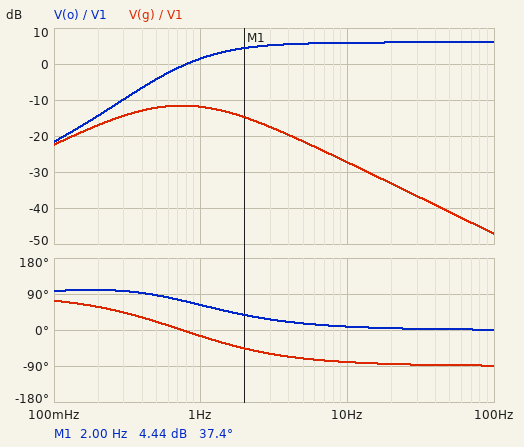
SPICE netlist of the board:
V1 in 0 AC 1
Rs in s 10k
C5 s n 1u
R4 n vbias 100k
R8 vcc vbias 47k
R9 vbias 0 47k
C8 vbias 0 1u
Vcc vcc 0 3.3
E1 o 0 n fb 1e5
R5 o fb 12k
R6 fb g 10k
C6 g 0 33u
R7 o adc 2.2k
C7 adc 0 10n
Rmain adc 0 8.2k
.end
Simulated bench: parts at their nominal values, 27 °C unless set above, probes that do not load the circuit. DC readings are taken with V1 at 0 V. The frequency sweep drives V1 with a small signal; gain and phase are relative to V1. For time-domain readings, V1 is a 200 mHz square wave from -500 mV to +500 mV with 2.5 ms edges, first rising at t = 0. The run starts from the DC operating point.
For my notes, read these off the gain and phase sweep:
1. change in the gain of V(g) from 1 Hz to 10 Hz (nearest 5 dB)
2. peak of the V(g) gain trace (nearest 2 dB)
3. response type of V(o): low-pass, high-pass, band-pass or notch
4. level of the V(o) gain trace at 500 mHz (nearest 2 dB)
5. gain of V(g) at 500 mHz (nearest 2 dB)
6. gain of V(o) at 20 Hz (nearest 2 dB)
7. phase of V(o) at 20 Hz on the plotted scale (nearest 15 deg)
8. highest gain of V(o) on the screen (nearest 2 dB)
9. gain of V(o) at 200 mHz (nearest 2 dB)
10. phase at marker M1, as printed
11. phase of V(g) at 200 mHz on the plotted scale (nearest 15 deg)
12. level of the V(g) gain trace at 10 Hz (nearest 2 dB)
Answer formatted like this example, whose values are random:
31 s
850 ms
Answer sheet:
-15 dB
-12 dB
high-pass
-4 dB
-12 dB
6 dB
0 deg
6 dB
-14 dB
37.4 deg
60 deg
-28 dB
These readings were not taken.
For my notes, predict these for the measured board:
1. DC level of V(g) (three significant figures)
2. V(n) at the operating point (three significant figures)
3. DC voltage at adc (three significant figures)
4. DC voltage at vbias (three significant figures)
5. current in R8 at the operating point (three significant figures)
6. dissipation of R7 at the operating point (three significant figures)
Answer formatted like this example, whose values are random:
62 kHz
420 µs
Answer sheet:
1.65 V
1.65 V
1.30 V
1.65 V
35.1 µA
55.4 µW
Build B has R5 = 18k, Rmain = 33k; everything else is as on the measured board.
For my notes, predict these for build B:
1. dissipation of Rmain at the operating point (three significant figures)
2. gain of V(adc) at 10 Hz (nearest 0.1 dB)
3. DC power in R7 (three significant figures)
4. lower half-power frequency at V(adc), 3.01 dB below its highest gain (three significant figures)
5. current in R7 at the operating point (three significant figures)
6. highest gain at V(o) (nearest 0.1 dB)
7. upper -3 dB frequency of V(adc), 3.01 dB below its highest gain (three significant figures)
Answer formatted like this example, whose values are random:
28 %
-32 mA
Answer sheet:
72.5 µW
7.4 dB
4.83 µW
1.34 Hz
46.9 µA
8.1 dB
7.72 kHz
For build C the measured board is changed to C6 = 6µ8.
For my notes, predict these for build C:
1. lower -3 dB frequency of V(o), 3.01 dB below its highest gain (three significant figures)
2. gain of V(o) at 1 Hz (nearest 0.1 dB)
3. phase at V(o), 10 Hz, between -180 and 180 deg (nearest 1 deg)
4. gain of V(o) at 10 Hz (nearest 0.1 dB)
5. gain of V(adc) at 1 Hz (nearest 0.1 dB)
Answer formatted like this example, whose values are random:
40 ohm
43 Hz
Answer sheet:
2.49 Hz
-2.6 dB
14 deg
5.7 dB
-4.7 dB
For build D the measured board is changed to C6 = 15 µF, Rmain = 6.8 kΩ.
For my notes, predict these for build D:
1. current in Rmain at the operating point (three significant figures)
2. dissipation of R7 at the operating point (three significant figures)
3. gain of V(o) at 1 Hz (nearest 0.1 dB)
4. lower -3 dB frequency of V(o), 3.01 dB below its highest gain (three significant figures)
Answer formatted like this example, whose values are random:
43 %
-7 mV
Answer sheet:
183 µA
73.9 µW
-0.2 dB
1.65 Hz
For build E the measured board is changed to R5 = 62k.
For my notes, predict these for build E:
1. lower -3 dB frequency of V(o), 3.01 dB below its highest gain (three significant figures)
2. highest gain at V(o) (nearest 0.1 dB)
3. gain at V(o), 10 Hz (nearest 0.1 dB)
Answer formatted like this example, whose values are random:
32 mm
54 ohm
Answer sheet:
1.36 Hz
16.3 dB
16.2 dB
